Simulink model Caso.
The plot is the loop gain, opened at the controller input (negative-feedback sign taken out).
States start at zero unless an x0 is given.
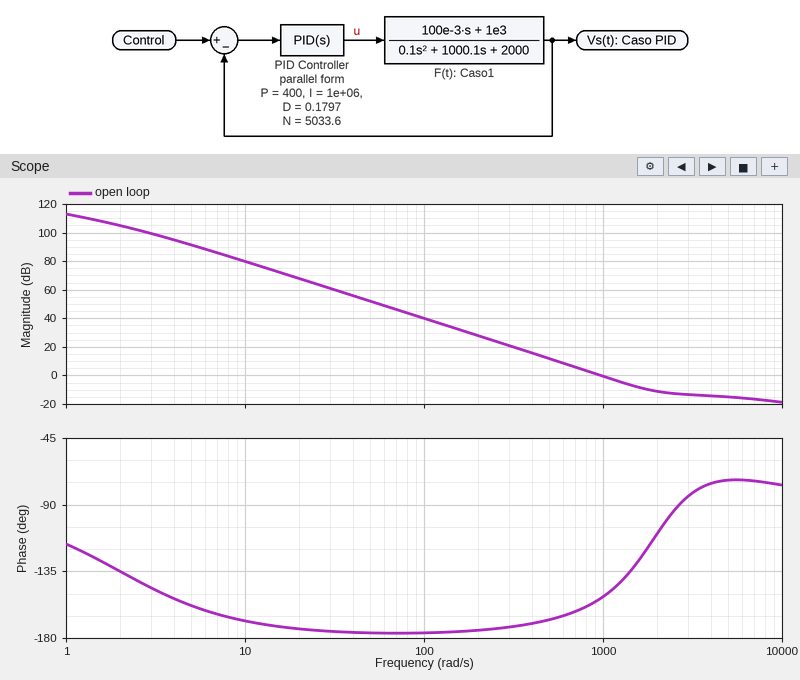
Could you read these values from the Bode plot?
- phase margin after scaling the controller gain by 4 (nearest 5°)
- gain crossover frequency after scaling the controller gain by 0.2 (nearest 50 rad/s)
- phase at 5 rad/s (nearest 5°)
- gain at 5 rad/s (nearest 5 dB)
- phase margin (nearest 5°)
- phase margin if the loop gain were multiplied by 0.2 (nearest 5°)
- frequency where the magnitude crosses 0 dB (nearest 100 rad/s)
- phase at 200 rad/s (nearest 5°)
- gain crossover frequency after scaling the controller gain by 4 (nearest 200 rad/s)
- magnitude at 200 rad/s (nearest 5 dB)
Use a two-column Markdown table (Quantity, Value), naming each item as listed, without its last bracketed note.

| Quantity | Value |
|---|---|
| phase margin after scaling the controller gain by 4 | 80° |
| gain crossover frequency after scaling the controller gain by 0.2 | 450 rad/s |
| phase at 5 rad/s | -160° |
| gain at 5 rad/s | 90 dB |
| phase margin | 25° |
| phase margin if the loop gain were multiplied by 0.2 | 10° |
| frequency where the magnitude crosses 0 dB | 1000 rad/s |
| phase at 200 rad/s | -175° |
| gain crossover frequency after scaling the controller gain by 4 | 2200 rad/s |
| magnitude at 200 rad/s | 30 dB |
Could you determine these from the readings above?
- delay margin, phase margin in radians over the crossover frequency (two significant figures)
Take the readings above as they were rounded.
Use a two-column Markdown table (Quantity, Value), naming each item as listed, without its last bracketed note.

| Quantity | Value |
|---|---|
| delay margin, phase margin in radians over the crossover frequency | 0.00044 s |
